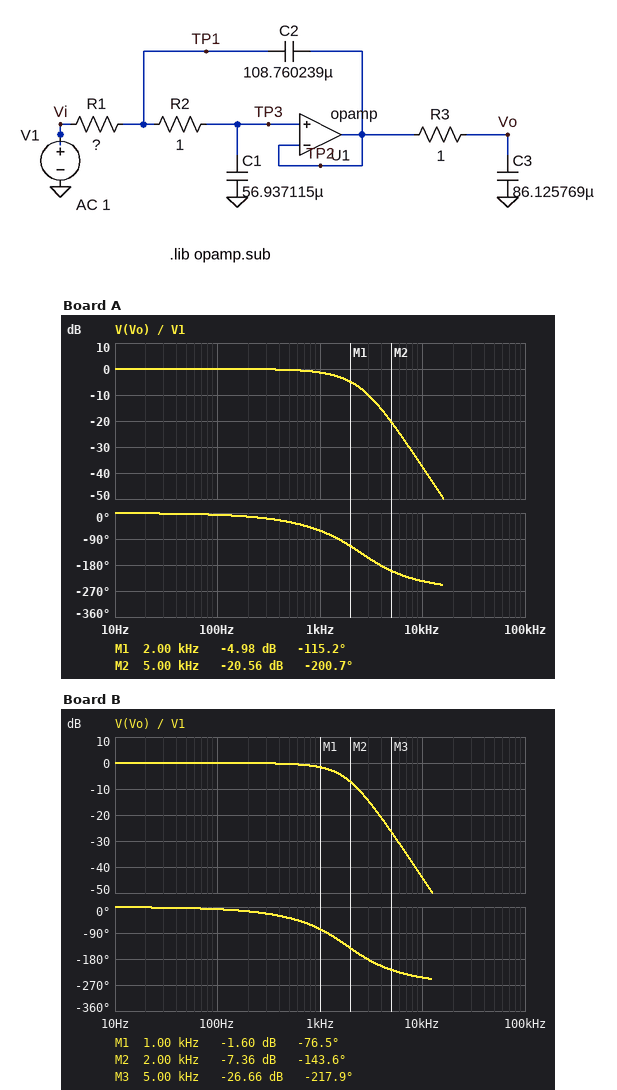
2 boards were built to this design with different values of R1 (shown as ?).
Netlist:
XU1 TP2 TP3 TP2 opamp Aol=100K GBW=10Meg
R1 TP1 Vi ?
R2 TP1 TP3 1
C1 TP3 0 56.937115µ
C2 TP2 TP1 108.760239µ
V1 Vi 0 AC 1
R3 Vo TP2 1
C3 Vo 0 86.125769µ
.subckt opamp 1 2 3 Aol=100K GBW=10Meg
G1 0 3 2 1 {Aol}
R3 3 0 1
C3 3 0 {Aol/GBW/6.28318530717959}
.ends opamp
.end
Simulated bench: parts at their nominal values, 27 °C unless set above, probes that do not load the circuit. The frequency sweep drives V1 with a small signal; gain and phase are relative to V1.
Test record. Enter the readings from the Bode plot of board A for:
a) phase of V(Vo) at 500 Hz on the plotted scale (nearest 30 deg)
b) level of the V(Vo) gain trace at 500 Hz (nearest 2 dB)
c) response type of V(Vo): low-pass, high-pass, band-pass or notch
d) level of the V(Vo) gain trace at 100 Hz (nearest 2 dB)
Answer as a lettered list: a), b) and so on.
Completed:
a) -30 deg
b) 0 dB
c) low-pass
d) 0 dB
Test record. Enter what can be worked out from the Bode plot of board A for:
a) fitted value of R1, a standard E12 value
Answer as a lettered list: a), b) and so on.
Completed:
a) 0.56 Ω
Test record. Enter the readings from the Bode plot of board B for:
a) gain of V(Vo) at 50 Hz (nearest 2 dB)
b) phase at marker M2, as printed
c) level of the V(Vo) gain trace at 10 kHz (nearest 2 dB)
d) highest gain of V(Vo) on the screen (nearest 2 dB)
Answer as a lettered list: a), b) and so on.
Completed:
a) 0 dB
b) -143.6 deg
c) -44 dB
d) 0 dB
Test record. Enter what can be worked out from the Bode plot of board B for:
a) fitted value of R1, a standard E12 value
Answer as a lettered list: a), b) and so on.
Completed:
a) 1.2 Ω
